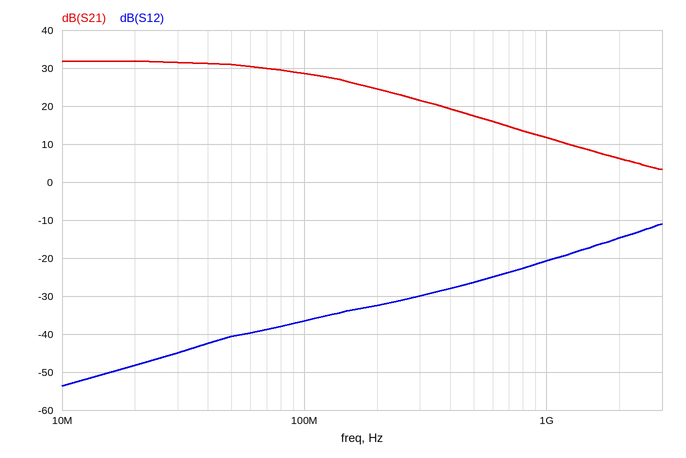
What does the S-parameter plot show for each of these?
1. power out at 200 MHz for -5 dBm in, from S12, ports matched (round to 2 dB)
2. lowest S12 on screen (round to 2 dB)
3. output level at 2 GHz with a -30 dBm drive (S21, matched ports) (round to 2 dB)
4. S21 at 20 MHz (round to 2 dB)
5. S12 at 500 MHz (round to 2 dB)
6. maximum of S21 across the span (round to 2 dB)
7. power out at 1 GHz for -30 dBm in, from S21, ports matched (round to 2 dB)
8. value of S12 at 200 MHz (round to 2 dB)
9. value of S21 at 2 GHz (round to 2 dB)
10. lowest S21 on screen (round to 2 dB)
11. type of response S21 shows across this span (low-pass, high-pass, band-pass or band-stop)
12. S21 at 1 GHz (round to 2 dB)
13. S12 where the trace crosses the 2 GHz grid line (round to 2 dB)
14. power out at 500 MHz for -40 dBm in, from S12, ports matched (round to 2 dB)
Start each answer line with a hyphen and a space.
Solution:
- -38 dBm
- -54 dB
- -24 dBm
- 32 dB
- -26 dB
- 32 dB
- -18 dBm
- -32 dB
- 6 dB
- 4 dB
- low-pass
- 12 dB
- -14 dB
- -66 dBm
